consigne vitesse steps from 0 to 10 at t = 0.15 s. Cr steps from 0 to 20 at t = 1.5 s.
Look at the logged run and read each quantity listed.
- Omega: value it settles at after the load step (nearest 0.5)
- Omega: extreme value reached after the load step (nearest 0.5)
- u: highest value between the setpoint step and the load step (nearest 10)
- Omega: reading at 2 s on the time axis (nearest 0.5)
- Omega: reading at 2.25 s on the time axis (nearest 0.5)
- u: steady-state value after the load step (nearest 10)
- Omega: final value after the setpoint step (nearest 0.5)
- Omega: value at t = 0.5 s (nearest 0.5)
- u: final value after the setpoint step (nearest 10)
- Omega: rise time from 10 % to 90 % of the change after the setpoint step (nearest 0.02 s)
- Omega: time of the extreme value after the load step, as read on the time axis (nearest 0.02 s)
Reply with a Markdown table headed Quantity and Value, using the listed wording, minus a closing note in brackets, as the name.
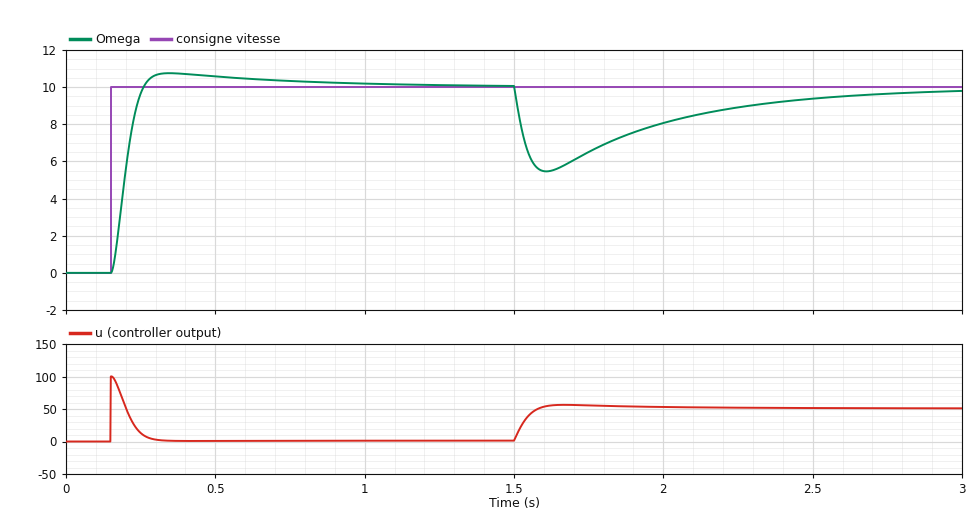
| Quantity | Value |
|---|---|
| Omega: value it settles at after the load step | 10.0 |
| Omega: extreme value reached after the load step | 5.5 |
| u: highest value between the setpoint step and the load step | 100 |
| Omega: reading at 2 s on the time axis | 8.0 |
| Omega: reading at 2.25 s on the time axis | 9.0 |
| u: steady-state value after the load step | 50 |
| Omega: final value after the setpoint step | 10.0 |
| Omega: value at t = 0.5 s | 10.5 |
| u: final value after the setpoint step | 0 |
| Omega: rise time from 10 % to 90 % of the change after the setpoint step | 0.08 s |
| Omega: time of the extreme value after the load step, as read on the time axis | 1.60 s |
